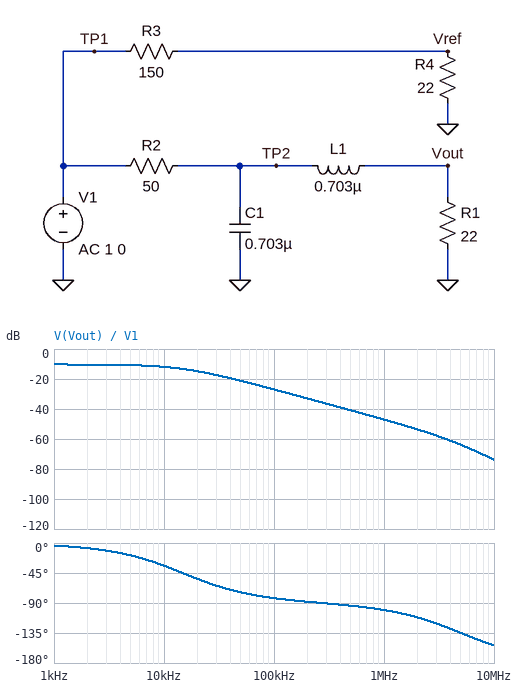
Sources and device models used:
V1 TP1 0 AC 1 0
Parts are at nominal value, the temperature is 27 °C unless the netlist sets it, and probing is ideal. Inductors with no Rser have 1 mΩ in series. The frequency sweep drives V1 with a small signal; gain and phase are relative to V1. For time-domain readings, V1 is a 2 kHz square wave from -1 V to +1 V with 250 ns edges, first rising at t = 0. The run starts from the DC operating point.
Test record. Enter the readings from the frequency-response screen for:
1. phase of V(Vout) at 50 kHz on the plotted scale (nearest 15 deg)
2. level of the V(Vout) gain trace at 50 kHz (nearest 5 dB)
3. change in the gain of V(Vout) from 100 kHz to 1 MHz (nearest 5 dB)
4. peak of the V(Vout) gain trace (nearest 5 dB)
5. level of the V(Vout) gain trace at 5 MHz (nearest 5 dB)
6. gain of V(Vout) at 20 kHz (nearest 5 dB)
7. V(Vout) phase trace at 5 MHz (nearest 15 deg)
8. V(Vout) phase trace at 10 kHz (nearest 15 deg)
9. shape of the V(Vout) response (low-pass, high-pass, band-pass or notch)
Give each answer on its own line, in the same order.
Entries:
-75 deg
-20 dB
-20 dB
-10 dB
-65 dB
-15 dB
-135 deg
-30 deg
low-pass
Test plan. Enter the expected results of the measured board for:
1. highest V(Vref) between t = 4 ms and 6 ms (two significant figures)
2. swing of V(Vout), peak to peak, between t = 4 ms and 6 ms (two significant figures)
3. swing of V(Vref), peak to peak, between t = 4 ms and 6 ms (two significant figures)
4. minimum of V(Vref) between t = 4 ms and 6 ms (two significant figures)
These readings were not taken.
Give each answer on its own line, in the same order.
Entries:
130 mV
610 mV
260 mV
-130 mV
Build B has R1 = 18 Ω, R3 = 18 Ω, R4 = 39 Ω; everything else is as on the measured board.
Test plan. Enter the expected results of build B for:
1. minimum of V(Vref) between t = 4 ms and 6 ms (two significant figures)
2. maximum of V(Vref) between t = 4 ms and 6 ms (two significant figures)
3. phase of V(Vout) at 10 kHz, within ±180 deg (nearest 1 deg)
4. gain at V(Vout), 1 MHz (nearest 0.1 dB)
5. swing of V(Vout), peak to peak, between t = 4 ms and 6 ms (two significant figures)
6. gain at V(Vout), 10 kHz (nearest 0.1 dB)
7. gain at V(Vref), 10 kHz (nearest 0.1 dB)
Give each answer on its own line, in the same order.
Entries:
-680 mV
680 mV
-30 deg
-47.1 dB
530 mV
-12.8 dB
-3.3 dB
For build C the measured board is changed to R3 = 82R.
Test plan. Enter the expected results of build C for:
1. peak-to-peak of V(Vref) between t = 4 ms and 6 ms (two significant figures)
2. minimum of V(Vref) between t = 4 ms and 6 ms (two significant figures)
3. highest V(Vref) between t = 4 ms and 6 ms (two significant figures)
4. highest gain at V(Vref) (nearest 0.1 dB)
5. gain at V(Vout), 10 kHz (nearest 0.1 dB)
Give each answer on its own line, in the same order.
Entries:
420 mV
-210 mV
210 mV
-13.5 dB
-11.9 dB
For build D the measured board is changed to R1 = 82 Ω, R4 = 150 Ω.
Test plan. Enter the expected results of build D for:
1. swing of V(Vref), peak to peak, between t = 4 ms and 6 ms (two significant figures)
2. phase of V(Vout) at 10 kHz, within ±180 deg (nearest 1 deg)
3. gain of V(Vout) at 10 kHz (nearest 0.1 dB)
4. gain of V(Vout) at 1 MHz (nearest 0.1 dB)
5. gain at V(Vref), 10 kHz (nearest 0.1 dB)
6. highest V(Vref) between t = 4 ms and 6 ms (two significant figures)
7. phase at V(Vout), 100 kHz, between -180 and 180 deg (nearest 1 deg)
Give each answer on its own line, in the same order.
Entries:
1.0 V
-54 deg
-8.7 dB
-46.9 dB
-6.0 dB
500 mV
-86 deg
